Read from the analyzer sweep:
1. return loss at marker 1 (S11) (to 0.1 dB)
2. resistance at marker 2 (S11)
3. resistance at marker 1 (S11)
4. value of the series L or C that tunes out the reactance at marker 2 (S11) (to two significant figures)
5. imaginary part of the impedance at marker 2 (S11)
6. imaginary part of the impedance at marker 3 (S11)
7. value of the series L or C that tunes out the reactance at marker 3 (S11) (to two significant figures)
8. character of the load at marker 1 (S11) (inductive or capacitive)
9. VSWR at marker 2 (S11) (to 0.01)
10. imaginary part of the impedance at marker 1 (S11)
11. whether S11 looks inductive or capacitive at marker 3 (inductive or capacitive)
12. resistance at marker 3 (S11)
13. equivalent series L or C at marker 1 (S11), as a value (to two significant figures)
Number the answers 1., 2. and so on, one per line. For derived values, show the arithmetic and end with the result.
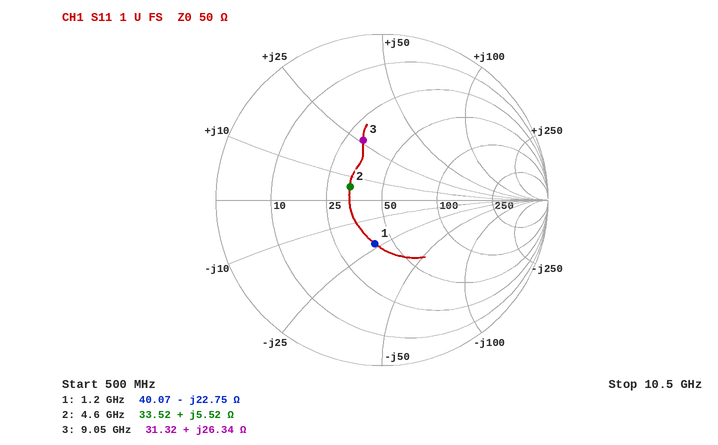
1. 11.5 dB
2. 33.52 Ω
3. 40.07 Ω
4. C = 1/(2π × 4.6 GHz × 5.52 Ω) ≈ 6.3 pF
5. +5.52 Ω
6. +26.34 Ω
7. C = 1/(2π × 9.05 GHz × 26.34 Ω) ≈ 668 fF, so 670 fF to two significant figures
8. capacitive
9. 1.52
10. -22.75 Ω
11. inductive
12. 31.32 Ω
13. C = 1/(2π × 1.2 GHz × 22.75 Ω) ≈ 5.8 pF
